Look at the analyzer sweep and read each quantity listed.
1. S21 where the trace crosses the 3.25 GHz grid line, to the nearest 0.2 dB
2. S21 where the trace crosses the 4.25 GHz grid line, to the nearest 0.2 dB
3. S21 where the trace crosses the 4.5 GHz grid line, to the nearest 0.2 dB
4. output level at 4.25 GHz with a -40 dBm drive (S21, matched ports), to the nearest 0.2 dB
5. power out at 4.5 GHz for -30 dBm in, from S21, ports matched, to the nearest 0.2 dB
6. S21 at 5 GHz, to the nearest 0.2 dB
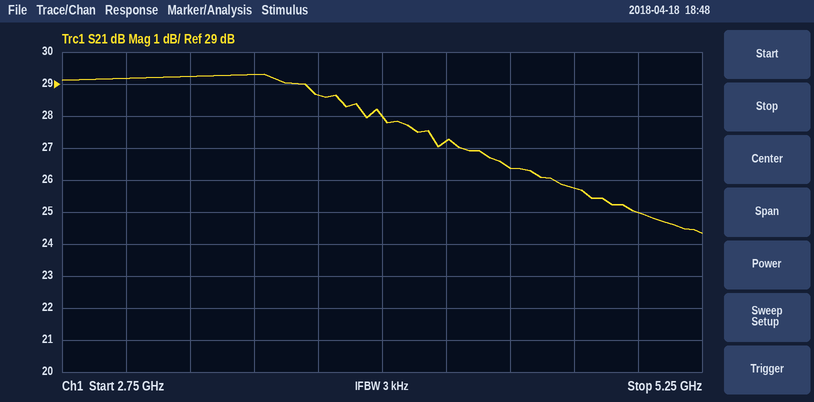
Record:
29.2 dB
27.2 dB
26.4 dB
-12.8 dBm
-3.6 dBm
25.0 dB
